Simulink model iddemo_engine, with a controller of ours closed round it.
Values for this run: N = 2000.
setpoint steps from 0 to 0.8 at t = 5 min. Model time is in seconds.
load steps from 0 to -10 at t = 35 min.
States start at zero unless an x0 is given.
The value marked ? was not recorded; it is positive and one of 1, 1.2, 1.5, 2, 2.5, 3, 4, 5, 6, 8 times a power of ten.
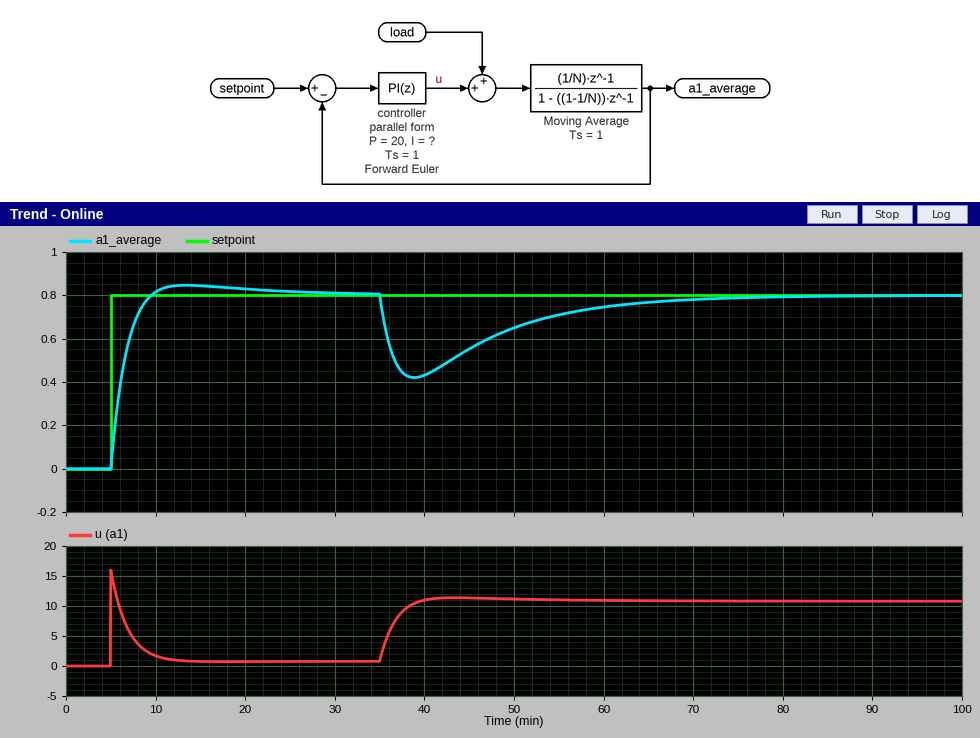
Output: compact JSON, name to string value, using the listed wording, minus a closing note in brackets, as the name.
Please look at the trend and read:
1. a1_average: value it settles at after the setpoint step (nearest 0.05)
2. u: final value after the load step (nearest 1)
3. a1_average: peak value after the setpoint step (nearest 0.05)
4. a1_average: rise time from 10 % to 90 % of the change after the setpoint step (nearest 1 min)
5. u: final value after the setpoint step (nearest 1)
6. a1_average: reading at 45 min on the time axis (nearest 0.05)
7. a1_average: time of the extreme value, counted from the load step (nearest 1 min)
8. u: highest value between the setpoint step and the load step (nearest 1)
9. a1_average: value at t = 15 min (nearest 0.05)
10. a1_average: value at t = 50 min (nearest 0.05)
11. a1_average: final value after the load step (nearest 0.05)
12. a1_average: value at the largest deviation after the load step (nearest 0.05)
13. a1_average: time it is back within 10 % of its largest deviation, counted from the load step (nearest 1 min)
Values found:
{"a1_average: value it settles at after the setpoint step": "0.80", "u: final value after the load step": "11", "a1_average: peak value after the setpoint step": "0.85", "a1_average: rise time from 10 % to 90 % of the change after the setpoint step": "3 min", "u: final value after the setpoint step": "1", "a1_average: reading at 45 min on the time axis": "0.55", "a1_average: time of the extreme value, counted from the load step": "4 min", "u: highest value between the setpoint step and the load step": "16", "a1_average: value at t = 15 min": "0.85", "a1_average: value at t = 50 min": "0.65", "a1_average: final value after the load step": "0.80", "a1_average: value at the largest deviation after the load step": "0.40", "a1_average: time it is back within 10 % of its largest deviation, counted from the load step": "28 min"}
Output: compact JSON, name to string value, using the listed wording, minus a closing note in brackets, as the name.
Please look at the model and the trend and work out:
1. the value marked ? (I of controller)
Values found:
{"the value marked ?": "0.03"}
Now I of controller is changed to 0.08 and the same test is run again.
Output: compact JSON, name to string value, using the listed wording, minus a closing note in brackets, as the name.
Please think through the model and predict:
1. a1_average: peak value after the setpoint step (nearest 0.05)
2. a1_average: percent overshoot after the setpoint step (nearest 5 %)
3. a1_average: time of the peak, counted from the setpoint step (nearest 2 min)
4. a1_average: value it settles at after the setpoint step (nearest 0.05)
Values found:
{"a1_average: peak value after the setpoint step": "0.90", "a1_average: percent overshoot after the setpoint step": "15 %", "a1_average: time of the peak, counted from the setpoint step": "6 min", "a1_average: value it settles at after the setpoint step": "0.80"}
